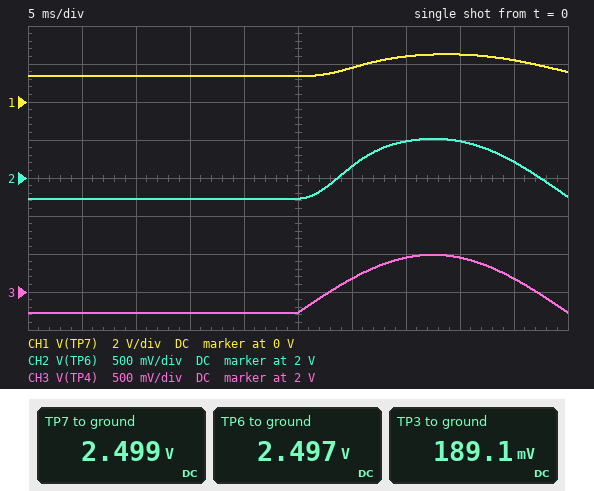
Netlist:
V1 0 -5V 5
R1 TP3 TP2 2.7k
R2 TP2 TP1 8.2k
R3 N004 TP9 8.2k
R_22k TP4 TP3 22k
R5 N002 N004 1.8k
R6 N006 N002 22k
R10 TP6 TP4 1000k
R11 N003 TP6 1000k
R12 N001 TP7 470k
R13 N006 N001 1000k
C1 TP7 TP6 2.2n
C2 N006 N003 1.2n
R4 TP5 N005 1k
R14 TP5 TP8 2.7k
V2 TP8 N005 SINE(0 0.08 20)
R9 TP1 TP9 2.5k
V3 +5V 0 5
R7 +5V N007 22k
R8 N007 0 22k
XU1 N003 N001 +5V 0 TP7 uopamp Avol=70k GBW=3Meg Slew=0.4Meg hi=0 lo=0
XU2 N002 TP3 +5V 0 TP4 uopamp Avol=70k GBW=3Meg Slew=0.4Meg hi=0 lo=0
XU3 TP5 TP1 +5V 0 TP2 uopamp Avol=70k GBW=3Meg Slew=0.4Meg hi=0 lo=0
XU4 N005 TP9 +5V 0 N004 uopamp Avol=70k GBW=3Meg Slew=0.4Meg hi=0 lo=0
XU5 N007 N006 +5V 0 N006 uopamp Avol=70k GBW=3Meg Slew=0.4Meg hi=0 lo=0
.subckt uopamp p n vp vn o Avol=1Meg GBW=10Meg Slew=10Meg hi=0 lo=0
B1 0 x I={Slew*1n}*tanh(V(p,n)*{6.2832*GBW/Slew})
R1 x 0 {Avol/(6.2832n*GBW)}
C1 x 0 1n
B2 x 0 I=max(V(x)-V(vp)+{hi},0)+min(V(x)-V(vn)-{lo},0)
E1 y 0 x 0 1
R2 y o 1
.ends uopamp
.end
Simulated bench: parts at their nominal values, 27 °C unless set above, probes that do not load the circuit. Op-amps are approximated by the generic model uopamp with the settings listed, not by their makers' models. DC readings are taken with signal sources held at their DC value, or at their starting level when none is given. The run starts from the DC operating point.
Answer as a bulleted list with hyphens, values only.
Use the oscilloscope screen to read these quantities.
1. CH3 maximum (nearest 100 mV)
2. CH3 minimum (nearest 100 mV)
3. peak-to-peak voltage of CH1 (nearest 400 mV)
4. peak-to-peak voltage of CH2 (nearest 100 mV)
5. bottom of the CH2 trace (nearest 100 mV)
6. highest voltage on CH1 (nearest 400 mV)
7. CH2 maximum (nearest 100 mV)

- 2.5 V
- 1.7 V
- 1.2 V
- 800 mV
- 1.7 V
- 2.4 V
- 2.5 V
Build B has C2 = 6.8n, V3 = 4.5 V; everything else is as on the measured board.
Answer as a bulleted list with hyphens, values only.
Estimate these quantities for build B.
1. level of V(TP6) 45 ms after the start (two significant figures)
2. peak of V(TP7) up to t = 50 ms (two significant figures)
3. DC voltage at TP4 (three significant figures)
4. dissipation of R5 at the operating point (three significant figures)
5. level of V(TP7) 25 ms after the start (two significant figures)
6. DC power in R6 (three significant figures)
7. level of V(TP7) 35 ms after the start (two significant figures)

- 2.1 V
- 2.0 V
- 1.56 V
- 16.1 µW
- 1.2 V
- 197 µW
- 1.6 V
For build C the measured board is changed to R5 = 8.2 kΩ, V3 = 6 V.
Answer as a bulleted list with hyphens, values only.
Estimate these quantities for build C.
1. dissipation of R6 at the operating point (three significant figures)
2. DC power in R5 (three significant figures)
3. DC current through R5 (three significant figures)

- 217 µW
- 80.9 µW
- 99.3 µA
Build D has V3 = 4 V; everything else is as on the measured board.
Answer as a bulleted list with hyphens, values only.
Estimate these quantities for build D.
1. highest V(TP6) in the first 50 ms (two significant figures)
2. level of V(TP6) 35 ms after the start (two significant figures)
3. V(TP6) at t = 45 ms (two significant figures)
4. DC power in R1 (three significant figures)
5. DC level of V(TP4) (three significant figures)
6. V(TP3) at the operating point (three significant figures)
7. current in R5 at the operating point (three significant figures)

- 2.2 V
- 2.1 V
- 1.9 V
- 8.47 µW
- 1.38 V
- 151 mV
- 84.0 µA
